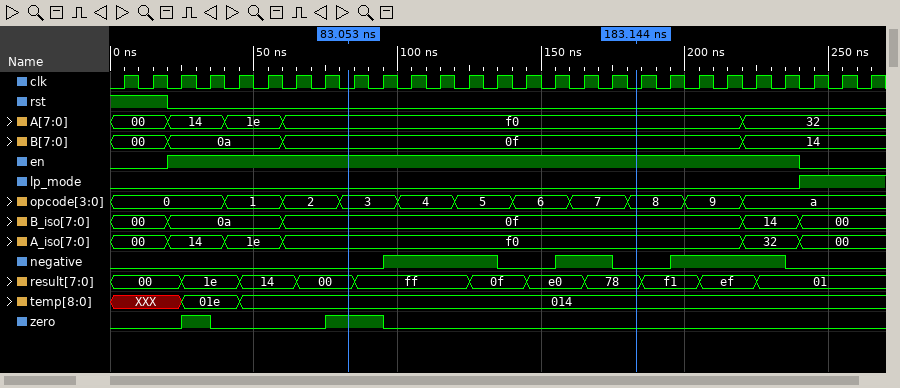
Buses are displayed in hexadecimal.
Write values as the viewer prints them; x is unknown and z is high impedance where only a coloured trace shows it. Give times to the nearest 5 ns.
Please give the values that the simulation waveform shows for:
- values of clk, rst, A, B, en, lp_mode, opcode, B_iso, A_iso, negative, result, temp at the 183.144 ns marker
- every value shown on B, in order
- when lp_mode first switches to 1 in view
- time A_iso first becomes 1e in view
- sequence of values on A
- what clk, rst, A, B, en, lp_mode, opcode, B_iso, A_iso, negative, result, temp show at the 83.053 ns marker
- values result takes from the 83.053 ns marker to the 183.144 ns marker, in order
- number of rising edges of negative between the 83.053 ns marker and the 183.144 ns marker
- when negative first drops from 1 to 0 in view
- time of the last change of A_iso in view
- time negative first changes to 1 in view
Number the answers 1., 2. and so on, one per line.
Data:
1. clk=0, rst=0, A=f0, B=0f, en=1, lp_mode=0, opcode=8, B_iso=0f, A_iso=f0, negative=0, result=78, temp=014
2. 00, 0a, 0f, 14
3. 240 ns
4. 40 ns
5. 00, 14, 1e, f0, 32
6. clk=0, rst=0, A=f0, B=0f, en=1, lp_mode=0, opcode=3, B_iso=0f, A_iso=f0, negative=0, result=00, temp=014
7. 00, ff, 0f, e0, 78
8. 2
9. 135 ns
10. 240 ns
11. 95 ns
